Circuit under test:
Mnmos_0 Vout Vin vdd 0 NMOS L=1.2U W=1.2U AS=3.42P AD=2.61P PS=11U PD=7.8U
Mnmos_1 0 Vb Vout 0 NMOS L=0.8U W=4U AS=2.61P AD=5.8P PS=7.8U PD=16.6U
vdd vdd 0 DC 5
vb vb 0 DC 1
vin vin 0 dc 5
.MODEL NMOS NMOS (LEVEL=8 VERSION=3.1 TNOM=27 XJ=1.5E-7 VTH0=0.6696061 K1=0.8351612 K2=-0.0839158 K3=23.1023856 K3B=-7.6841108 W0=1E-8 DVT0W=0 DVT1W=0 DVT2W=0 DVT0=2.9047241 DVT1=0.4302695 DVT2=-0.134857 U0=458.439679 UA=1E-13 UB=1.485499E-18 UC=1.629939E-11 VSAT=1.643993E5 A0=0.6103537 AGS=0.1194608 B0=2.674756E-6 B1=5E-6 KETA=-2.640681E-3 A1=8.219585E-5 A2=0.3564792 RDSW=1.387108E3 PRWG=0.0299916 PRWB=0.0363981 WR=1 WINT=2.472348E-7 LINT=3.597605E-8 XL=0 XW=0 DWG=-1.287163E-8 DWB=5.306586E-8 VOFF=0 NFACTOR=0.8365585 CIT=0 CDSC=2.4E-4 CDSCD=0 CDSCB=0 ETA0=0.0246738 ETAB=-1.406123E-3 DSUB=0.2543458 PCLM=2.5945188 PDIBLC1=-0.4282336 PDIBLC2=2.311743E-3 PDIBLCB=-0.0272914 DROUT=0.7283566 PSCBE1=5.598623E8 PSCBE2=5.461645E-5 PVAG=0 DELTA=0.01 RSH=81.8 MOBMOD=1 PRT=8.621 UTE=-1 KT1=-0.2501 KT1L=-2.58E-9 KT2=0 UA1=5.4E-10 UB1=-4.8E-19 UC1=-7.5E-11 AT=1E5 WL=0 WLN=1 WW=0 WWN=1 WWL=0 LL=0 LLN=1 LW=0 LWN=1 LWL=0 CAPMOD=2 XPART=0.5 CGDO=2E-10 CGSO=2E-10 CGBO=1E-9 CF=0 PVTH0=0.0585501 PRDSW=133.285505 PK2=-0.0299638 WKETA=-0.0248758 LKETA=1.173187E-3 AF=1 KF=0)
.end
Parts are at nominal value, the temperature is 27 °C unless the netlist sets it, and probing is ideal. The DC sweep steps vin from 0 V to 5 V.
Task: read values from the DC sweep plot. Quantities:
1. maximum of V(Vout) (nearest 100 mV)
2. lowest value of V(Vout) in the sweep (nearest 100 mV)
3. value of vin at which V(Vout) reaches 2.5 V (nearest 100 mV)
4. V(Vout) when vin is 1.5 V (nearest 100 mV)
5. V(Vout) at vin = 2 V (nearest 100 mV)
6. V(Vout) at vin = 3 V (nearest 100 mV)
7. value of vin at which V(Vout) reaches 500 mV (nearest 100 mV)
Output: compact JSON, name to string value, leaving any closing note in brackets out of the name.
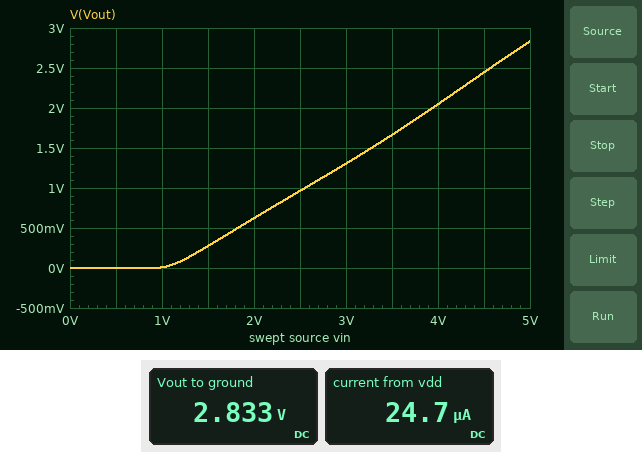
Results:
{"maximum of V(Vout)": "2.8 V", "lowest value of V(Vout) in the sweep": "0 V", "value of vin at which V(Vout) reaches 2.5 V": "4.6 V", "V(Vout) when vin is 1.5 V": "300 mV", "V(Vout) at vin = 2 V": "600 mV", "V(Vout) at vin = 3 V": "1.3 V", "value of vin at which V(Vout) reaches 500 mV": "1.8 V"}
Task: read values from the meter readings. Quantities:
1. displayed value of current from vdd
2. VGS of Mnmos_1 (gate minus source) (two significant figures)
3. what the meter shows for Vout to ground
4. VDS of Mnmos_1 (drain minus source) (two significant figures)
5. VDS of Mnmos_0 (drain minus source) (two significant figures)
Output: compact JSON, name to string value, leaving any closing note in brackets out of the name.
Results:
{"displayed value of current from vdd": "24.7 µA", "VGS of Mnmos_1 (gate minus source)": "-1.8 V", "what the meter shows for Vout to ground": "2.833 V", "VDS of Mnmos_1 (drain minus source)": "-2.8 V", "VDS of Mnmos_0 (drain minus source)": "-2.2 V"}
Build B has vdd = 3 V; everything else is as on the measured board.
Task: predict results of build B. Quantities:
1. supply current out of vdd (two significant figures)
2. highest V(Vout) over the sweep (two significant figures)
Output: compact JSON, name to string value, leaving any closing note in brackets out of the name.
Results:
{"supply current out of vdd": "23 µA", "highest V(Vout) over the sweep": "2.6 V"}
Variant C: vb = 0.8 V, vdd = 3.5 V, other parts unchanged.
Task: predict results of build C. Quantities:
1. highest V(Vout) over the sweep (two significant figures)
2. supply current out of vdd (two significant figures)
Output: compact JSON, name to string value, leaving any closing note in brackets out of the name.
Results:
{"highest V(Vout) over the sweep": "3.4 V", "supply current out of vdd": "230 nA"}
